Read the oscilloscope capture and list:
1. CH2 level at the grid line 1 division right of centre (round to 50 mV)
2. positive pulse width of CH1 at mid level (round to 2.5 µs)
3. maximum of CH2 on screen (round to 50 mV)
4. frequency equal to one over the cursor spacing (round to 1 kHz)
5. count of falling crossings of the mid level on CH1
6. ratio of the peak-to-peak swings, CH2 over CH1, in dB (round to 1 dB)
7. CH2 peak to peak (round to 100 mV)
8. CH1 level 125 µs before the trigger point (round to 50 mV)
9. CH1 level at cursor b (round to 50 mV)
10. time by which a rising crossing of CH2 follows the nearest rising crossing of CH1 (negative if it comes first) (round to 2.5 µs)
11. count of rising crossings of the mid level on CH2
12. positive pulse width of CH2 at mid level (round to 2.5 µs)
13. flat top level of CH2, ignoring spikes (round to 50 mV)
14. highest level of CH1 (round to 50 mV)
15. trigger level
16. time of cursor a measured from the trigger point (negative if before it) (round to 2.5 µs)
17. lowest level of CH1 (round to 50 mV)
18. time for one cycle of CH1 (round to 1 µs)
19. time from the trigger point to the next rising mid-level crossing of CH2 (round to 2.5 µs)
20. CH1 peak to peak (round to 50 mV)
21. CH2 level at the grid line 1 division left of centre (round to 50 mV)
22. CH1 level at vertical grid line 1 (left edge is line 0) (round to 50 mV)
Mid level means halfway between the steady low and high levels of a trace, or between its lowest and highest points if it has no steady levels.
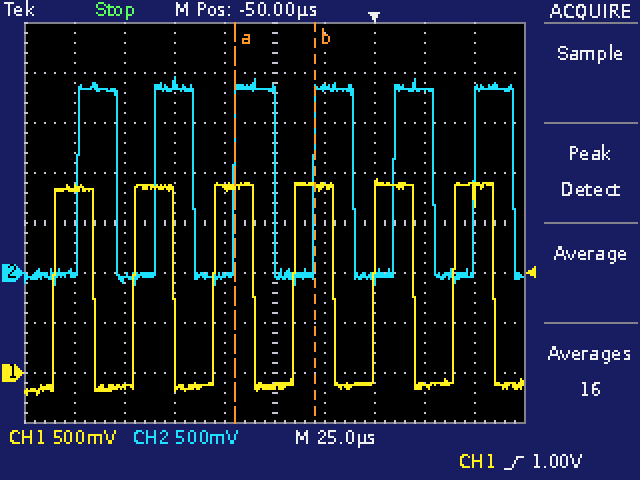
1.85 V
20.0 µs
1.95 V
25 kHz
6
0 dB
2.10 V
-150 mV
1.85 V
+10.0 µs
6
20.0 µs
1.85 V
1.95 V
1.00 V
-70.0 µs
-200 mV
40 µs
10.0 µs
2.15 V
-50 mV
1.85 V
